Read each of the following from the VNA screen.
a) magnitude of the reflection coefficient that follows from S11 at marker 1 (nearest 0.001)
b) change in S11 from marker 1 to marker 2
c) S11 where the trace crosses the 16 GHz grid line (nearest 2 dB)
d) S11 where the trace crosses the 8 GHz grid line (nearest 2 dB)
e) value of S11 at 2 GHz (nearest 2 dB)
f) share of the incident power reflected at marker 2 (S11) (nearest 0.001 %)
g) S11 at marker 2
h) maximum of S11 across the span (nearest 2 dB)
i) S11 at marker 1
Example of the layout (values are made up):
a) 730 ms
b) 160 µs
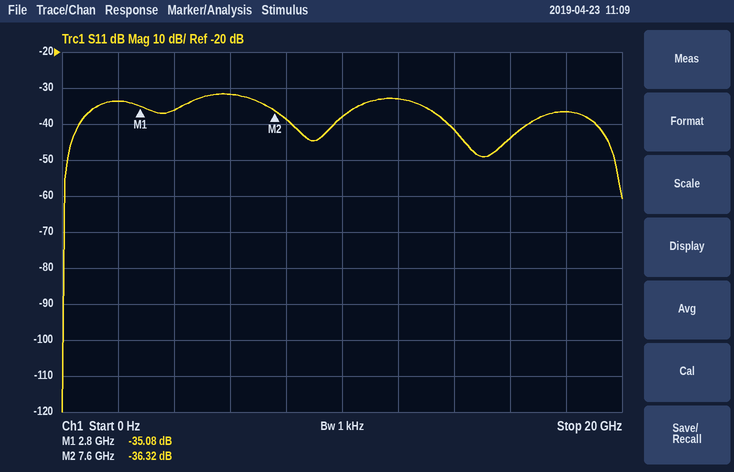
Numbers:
a) 0.018
b) -1.24 dB
c) -44 dB
d) -38 dB
e) -34 dB
f) 0.023 %
g) -36.32 dB
h) -32 dB
i) -35.08 dB
